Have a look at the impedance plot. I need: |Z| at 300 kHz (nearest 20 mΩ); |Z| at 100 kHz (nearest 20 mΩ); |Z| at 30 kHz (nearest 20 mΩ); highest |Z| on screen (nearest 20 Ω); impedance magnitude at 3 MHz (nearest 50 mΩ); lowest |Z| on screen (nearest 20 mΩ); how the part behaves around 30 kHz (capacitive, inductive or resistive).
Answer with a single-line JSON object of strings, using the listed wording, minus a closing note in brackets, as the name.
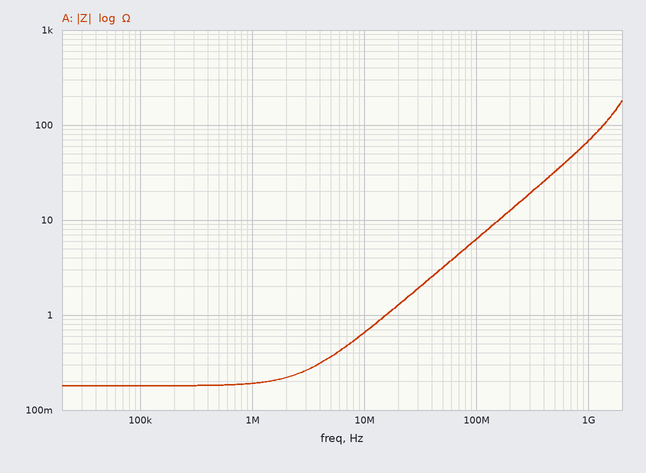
{"|Z| at 300 kHz": "180 mΩ", "|Z| at 100 kHz": "180 mΩ", "|Z| at 30 kHz": "180 mΩ", "highest |Z| on screen": "180 Ω", "impedance magnitude at 3 MHz": "250 mΩ", "lowest |Z| on screen": "180 mΩ", "how the part behaves around 30 kHz": "resistive"}
